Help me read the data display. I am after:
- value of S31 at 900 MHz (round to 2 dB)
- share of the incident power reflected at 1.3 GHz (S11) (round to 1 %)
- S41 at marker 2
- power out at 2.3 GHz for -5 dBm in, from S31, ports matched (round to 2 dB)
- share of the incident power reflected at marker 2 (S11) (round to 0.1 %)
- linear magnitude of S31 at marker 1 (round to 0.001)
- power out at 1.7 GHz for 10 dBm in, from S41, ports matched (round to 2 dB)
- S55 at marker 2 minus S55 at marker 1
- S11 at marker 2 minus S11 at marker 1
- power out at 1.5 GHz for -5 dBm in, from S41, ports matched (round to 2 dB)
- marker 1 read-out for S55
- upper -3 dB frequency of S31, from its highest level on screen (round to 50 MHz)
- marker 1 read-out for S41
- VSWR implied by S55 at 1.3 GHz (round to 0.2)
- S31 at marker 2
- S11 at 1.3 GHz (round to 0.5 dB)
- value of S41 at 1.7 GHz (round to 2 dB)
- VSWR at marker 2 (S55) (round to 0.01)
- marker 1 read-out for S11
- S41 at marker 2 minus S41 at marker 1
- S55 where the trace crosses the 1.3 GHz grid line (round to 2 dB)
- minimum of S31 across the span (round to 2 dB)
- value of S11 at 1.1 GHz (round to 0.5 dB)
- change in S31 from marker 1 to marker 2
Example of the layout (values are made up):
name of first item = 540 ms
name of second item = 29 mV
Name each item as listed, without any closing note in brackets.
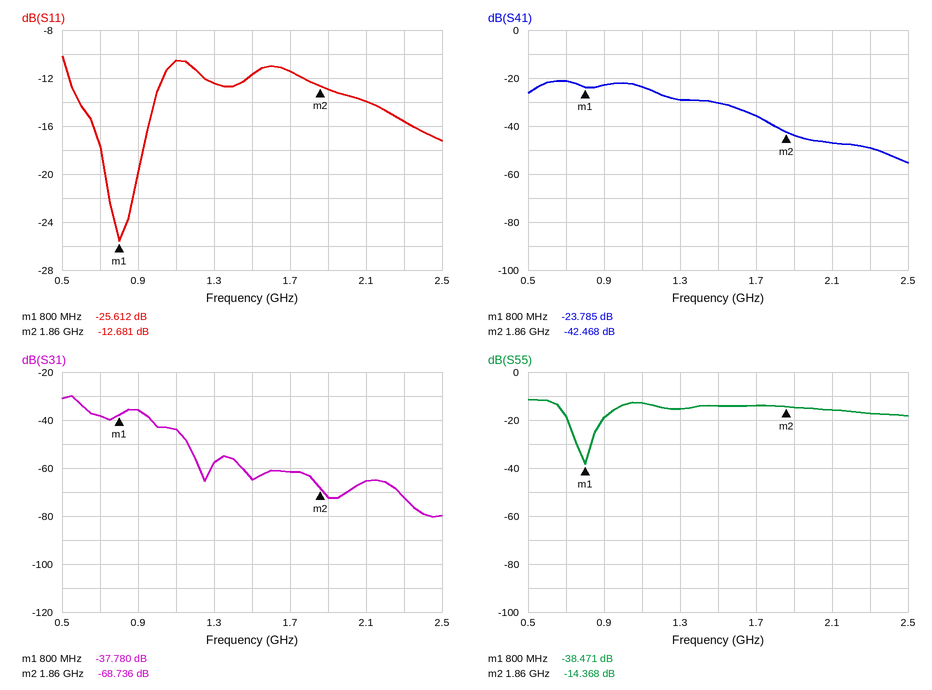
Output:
value of S31 at 900 MHz = -36 dB
share of the incident power reflected at 1.3 GHz (S11) = 6 %
S41 at marker 2 = -42.468 dB
power out at 2.3 GHz for -5 dBm in, from S31, ports matched = -78 dBm
share of the incident power reflected at marker 2 (S11) = 5.4 %
linear magnitude of S31 at marker 1 = 0.013
power out at 1.7 GHz for 10 dBm in, from S41, ports matched = -26 dBm
S55 at marker 2 minus S55 at marker 1 = 24.103 dB
S11 at marker 2 minus S11 at marker 1 = 12.931 dB
power out at 1.5 GHz for -5 dBm in, from S41, ports matched = -36 dBm
marker 1 read-out for S55 = -38.471 dB
upper -3 dB frequency of S31, from its highest level on screen = 600 MHz
marker 1 read-out for S41 = -23.785 dB
VSWR implied by S55 at 1.3 GHz = 1.4
S31 at marker 2 = -68.736 dB
S11 at 1.3 GHz = -12.5 dB
value of S41 at 1.7 GHz = -36 dB
VSWR at marker 2 (S55) = 1.47
marker 1 read-out for S11 = -25.612 dB
S41 at marker 2 minus S41 at marker 1 = -18.683 dB
S55 where the trace crosses the 1.3 GHz grid line = -16 dB
minimum of S31 across the span = -80 dB
value of S11 at 1.1 GHz = -10.5 dB
change in S31 from marker 1 to marker 2 = -30.956 dB
